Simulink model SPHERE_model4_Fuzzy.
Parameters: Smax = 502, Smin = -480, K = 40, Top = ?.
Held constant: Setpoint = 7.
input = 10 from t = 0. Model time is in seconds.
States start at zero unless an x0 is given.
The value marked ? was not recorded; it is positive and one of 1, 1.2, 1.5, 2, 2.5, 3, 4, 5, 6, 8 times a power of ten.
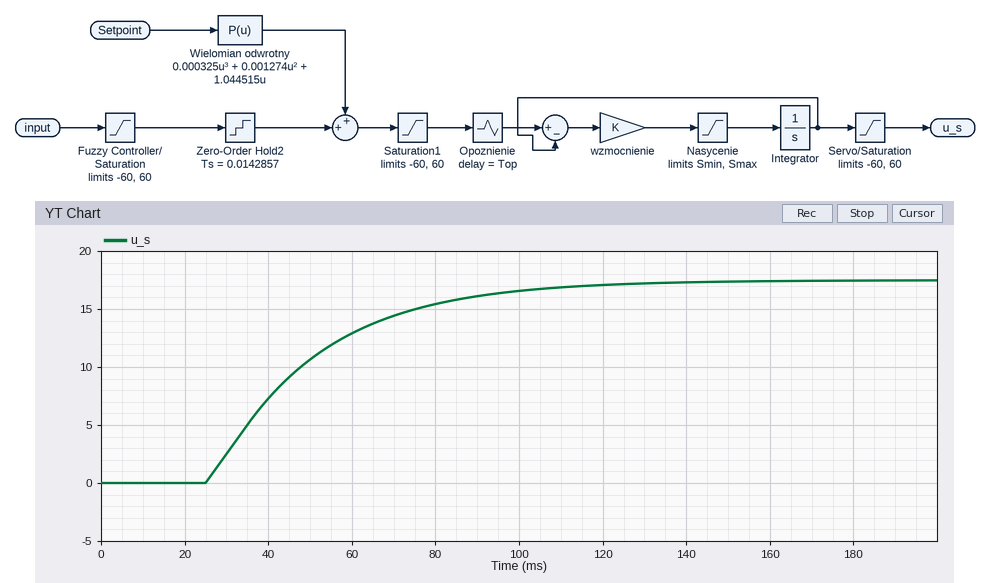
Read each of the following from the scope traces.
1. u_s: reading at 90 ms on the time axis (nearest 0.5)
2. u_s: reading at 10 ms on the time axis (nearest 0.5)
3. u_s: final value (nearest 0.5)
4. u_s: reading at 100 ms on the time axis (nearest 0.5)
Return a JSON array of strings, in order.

["16.0", "0.0", "17.5", "16.5"]
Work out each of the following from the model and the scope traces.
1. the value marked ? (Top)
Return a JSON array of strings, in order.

["0.025"]
